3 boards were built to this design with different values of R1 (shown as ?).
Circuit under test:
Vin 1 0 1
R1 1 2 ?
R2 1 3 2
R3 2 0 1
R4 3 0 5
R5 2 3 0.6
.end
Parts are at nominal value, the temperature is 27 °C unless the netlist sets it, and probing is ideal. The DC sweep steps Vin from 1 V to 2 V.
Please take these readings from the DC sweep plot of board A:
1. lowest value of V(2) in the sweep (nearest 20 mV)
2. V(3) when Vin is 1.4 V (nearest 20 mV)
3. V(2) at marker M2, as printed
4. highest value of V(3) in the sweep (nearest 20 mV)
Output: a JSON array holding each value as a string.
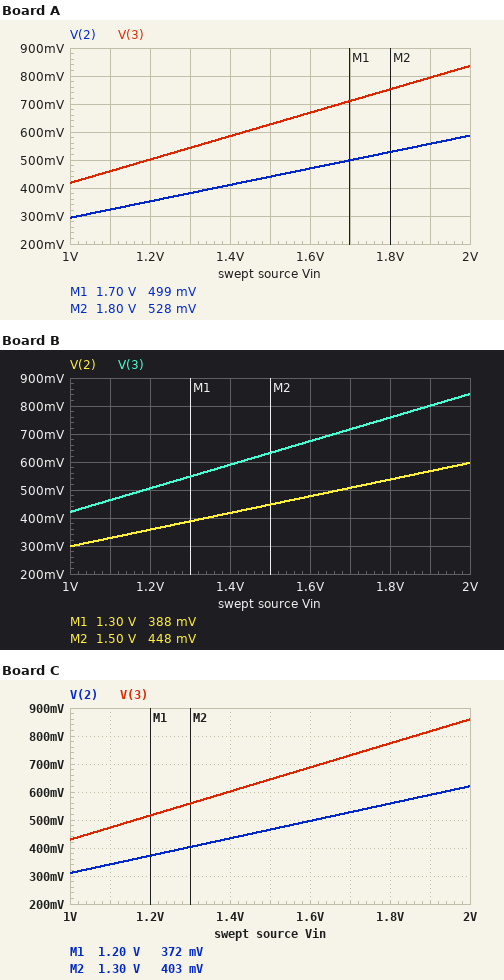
["300 mV", "580 mV", "528 mV", "840 mV"]
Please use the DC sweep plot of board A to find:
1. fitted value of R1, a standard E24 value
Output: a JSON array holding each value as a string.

["8.2 Ω"]
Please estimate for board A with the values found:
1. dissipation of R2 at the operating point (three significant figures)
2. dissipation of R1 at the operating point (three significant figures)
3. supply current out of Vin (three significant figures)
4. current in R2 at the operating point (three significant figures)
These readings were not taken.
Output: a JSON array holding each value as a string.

["169 mW", "60.9 mW", "377 mA", "291 mA"]
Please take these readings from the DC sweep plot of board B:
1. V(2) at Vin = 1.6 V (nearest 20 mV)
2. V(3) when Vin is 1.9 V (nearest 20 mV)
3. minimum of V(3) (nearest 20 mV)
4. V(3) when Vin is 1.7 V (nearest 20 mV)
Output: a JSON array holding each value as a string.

["480 mV", "800 mV", "420 mV", "720 mV"]
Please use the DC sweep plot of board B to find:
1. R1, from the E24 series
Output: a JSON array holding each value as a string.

["7.5 Ω"]
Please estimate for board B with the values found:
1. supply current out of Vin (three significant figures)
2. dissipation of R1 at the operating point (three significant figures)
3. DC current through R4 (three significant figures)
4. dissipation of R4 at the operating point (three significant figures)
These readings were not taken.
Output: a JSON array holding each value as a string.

["383 mA", "65.6 mW", "84.3 mA", "35.5 mW"]
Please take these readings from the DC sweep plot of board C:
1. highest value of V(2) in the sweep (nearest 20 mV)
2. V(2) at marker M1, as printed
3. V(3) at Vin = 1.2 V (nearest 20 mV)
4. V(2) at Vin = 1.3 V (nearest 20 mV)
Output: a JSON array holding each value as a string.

["620 mV", "372 mV", "520 mV", "400 mV"]
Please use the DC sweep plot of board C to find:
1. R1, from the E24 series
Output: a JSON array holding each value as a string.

["6.2 Ω"]
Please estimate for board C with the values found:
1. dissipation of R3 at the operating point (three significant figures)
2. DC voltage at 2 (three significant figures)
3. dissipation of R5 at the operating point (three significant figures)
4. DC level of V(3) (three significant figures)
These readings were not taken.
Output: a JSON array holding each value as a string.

["96.3 mW", "310 mV", "23.8 mW", "430 mV"]
